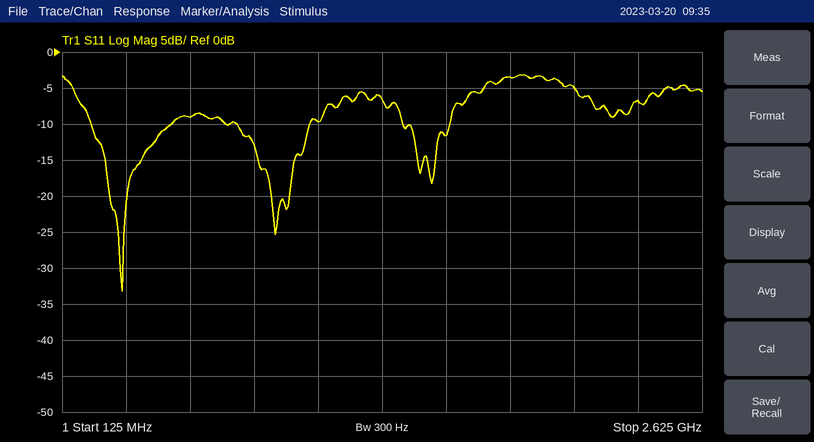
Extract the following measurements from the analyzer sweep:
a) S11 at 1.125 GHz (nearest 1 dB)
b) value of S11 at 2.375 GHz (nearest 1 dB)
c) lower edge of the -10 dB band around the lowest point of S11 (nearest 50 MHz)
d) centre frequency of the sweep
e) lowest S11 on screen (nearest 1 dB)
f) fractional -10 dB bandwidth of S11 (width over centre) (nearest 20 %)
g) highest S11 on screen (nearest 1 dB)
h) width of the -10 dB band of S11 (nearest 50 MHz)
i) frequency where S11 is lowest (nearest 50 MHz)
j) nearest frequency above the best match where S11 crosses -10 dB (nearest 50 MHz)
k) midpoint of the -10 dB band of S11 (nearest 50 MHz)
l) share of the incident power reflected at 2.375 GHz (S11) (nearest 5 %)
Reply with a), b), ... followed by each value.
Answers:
a) -10 dB
b) -7 dB
c) 250 MHz
d) 1.375 GHz
e) -33 dB
f) 80 %
g) -3 dB
h) 300 MHz
i) 350 MHz
j) 550 MHz
k) 400 MHz
l) 20 %
